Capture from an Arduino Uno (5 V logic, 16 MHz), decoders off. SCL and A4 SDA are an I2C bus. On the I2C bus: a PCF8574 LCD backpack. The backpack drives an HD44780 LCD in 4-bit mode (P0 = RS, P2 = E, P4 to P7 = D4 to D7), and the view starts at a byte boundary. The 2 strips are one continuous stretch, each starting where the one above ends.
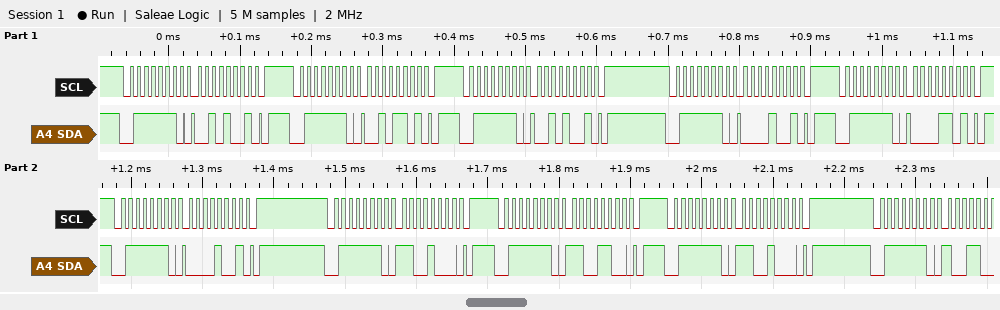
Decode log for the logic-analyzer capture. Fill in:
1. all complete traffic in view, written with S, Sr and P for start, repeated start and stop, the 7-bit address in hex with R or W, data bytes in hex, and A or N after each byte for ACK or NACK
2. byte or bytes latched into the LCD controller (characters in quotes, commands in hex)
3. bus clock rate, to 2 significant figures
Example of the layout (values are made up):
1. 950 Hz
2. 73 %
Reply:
1. S 3FW A 29 A P S 3FW A 2D A P S 3FW A 29 A P S 3FW A 09 A P S 3FW A 0D A P S 3FW A 09 A P S 3FW A C8 A P S 3FW A CC A P S 3FW A C8 A P S 3FW A
2. ' '
3. 100 kHz
